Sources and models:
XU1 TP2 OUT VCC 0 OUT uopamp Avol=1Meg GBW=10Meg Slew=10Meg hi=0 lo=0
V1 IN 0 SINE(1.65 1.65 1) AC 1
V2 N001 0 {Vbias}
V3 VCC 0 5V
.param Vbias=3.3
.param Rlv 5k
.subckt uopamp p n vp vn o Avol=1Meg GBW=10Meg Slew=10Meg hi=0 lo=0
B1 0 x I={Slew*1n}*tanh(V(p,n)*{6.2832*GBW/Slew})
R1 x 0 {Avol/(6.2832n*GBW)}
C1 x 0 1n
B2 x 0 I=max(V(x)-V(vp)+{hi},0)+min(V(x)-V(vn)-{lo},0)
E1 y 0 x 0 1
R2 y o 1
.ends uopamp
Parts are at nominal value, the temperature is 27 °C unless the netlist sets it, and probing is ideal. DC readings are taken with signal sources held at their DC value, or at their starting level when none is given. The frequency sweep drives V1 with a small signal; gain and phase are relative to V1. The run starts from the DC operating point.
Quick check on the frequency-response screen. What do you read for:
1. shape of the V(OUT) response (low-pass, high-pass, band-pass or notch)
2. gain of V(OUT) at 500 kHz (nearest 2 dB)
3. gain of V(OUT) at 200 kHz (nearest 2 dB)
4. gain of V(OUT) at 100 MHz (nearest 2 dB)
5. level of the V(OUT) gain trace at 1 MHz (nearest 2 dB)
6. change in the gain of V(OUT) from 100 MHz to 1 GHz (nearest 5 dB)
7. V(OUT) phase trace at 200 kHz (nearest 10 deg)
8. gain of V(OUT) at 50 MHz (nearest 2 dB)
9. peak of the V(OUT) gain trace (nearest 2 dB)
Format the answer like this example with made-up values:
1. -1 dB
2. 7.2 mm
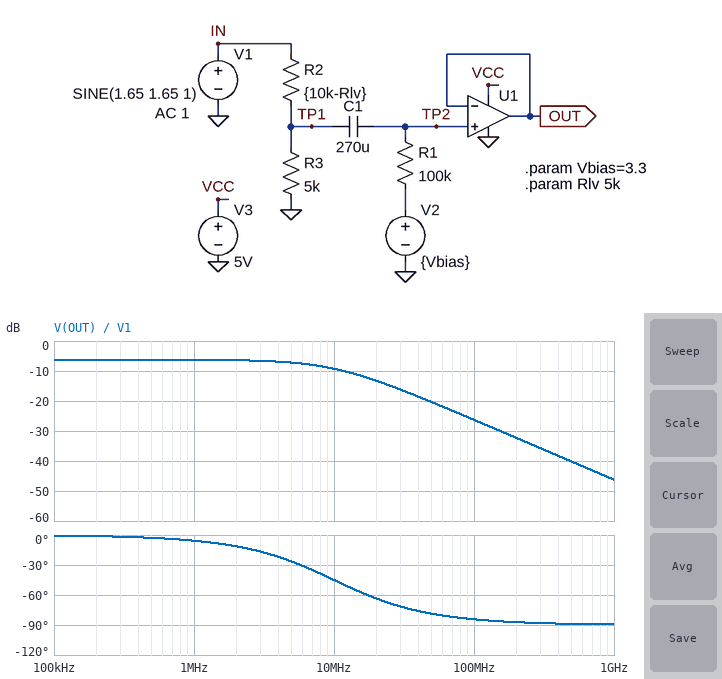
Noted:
1. low-pass
2. -6 dB
3. -6 dB
4. -26 dB
5. -6 dB
6. -20 dB
7. 0 deg
8. -20 dB
9. -6 dB
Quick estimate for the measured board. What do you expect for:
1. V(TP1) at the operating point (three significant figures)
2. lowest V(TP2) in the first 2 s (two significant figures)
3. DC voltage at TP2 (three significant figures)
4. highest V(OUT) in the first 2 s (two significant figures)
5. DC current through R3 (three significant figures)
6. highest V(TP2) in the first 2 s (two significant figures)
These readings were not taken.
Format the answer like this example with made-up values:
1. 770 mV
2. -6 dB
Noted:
1. 825 mV
2. 2.5 V
3. 3.30 V
4. 4.1 V
5. 165 µA
6. 4.1 V
